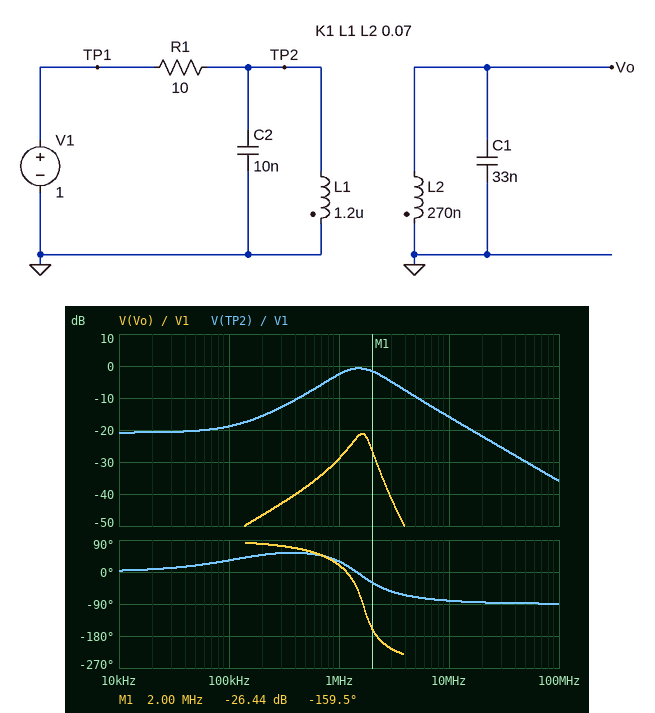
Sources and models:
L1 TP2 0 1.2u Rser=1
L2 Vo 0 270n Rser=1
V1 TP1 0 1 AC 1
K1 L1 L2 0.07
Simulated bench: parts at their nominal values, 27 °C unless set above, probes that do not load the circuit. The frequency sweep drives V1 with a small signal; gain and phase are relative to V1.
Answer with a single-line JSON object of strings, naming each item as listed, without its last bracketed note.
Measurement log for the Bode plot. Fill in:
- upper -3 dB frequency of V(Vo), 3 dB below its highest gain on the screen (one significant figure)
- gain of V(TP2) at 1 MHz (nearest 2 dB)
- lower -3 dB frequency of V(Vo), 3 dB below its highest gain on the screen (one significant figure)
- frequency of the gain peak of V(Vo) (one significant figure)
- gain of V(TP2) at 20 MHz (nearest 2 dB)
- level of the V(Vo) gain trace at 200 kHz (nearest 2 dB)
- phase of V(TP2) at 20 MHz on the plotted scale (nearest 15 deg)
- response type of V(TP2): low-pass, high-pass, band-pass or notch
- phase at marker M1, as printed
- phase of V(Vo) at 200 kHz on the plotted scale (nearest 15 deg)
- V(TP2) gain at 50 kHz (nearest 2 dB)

{"upper -3 dB frequency of V(Vo), 3 dB below its highest gain on the screen": "2 MHz", "gain of V(TP2) at 1 MHz": "-2 dB", "lower -3 dB frequency of V(Vo), 3 dB below its highest gain on the screen": "1 MHz", "frequency of the gain peak of V(Vo)": "2 MHz", "gain of V(TP2) at 20 MHz": "-22 dB", "level of the V(Vo) gain trace at 200 kHz": "-46 dB", "phase of V(TP2) at 20 MHz on the plotted scale": "-90 deg", "response type of V(TP2): low-pass, high-pass, band-pass or notch": "band-pass", "phase at marker M1, as printed": "-159.5 deg", "phase of V(Vo) at 200 kHz on the plotted scale": "75 deg", "V(TP2) gain at 50 kHz": "-20 dB"}
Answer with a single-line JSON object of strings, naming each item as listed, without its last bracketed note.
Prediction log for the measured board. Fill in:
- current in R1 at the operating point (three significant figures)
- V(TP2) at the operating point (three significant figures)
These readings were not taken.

{"current in R1 at the operating point": "90.9 mA", "V(TP2) at the operating point": "90.9 mV"}
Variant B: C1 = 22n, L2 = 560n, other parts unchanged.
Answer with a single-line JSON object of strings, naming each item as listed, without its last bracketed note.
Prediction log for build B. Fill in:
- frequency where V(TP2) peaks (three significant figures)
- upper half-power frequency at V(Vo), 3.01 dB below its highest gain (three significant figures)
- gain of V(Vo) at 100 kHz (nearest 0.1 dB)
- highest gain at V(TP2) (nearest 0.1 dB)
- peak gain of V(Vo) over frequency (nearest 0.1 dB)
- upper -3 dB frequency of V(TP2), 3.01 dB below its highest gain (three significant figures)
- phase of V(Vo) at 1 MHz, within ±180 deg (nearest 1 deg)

{"frequency where V(TP2) peaks": "1.58 MHz", "upper half-power frequency at V(Vo), 3.01 dB below its highest gain": "1.56 MHz", "gain of V(Vo) at 100 kHz": "-49.6 dB", "highest gain at V(TP2)": "-0.8 dB", "peak gain of V(Vo) over frequency": "-13.3 dB", "upper -3 dB frequency of V(TP2), 3.01 dB below its highest gain": "2.64 MHz", "phase of V(Vo) at 1 MHz, within ±180 deg": "22 deg"}
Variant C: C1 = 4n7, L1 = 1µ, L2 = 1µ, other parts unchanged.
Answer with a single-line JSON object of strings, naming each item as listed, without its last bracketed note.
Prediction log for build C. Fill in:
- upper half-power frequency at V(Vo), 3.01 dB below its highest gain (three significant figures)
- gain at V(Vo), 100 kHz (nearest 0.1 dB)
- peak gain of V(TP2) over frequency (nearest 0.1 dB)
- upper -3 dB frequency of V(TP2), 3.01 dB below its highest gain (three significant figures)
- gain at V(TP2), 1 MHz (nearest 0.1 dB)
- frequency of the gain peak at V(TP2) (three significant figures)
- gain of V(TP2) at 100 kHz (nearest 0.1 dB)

{"upper half-power frequency at V(Vo), 3.01 dB below its highest gain": "2.40 MHz", "gain at V(Vo), 100 kHz": "-47.9 dB", "peak gain of V(TP2) over frequency": "-0.8 dB", "upper -3 dB frequency of V(TP2), 3.01 dB below its highest gain": "2.76 MHz", "gain at V(TP2), 1 MHz": "-3.8 dB", "frequency of the gain peak at V(TP2)": "1.66 MHz", "gain of V(TP2) at 100 kHz": "-19.4 dB"}
